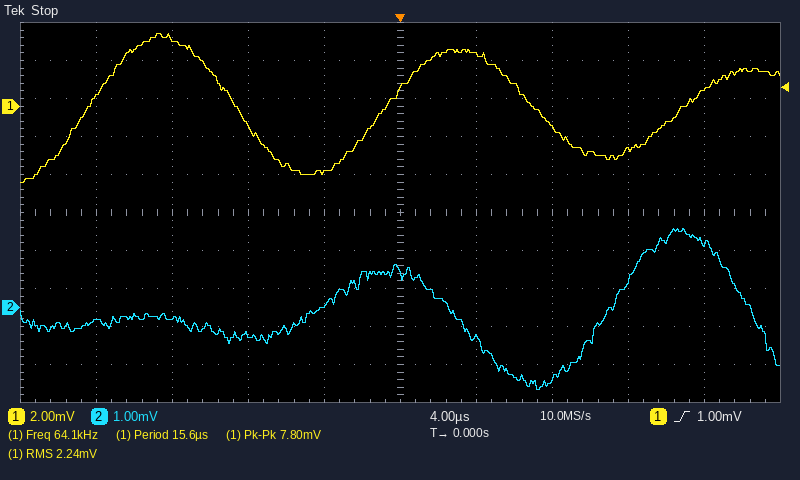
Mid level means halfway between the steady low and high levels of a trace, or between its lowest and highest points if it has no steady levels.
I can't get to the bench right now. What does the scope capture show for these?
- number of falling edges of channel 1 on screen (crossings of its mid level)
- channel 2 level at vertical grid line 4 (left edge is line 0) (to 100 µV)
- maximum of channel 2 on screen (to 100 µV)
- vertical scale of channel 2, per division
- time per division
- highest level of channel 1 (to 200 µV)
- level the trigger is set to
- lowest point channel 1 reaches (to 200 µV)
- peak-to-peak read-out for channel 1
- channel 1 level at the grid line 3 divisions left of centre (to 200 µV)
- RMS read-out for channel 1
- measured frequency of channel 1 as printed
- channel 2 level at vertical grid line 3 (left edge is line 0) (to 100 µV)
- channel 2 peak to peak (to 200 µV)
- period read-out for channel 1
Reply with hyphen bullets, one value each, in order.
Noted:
- 2
- 100 µV
- 2.1 mV
- 1 mV
- 4 µs
- 3.8 mV
- 1.00 mV
- -4.0 mV
- 7.80 mV
- 3.6 mV
- 2.24 mV
- 64.1 kHz
- -700 µV
- 4.2 mV
- 15.6 µs
